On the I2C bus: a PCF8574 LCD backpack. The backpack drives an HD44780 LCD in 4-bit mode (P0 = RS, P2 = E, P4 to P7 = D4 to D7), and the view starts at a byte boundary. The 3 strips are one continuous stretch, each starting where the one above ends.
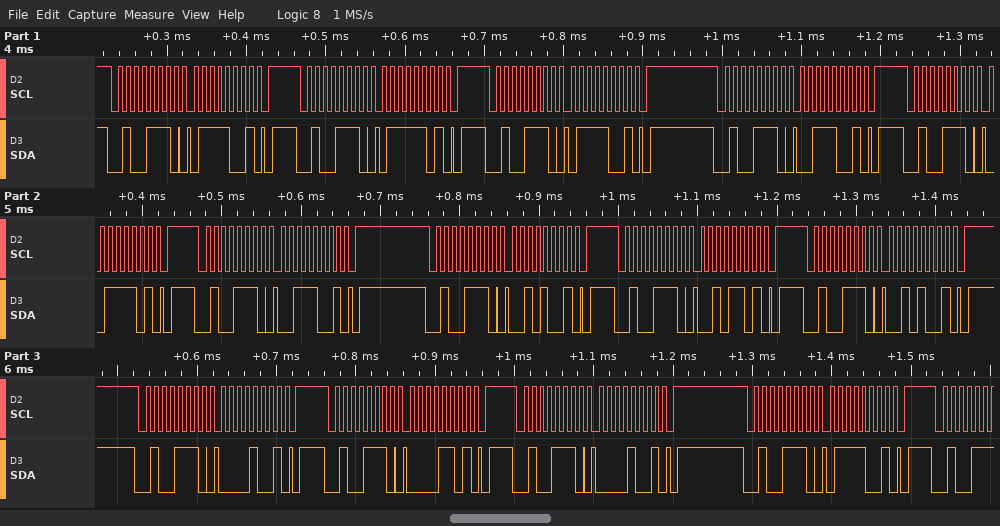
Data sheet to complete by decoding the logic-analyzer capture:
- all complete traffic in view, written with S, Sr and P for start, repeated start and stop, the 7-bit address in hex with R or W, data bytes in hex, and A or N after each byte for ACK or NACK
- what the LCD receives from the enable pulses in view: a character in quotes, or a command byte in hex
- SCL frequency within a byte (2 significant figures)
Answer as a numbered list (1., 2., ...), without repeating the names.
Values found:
1. S 27W A 79 A P S 27W A 7D A P S 27W A 79 A P S 27W A 39 A P S 27W A 3D A P S 27W A 39 A P S 27W A 29 A P S 27W A 2D A P S 27W A 29 A P S 27W A 09 A P S 27W A 0D A P S 27W A 09 A P S 27W A 79 A P
2. 's' ' '
3. 100 kHz
